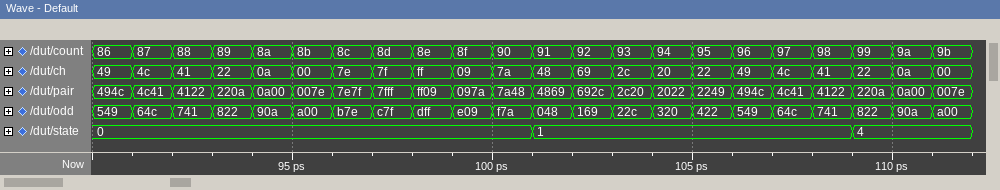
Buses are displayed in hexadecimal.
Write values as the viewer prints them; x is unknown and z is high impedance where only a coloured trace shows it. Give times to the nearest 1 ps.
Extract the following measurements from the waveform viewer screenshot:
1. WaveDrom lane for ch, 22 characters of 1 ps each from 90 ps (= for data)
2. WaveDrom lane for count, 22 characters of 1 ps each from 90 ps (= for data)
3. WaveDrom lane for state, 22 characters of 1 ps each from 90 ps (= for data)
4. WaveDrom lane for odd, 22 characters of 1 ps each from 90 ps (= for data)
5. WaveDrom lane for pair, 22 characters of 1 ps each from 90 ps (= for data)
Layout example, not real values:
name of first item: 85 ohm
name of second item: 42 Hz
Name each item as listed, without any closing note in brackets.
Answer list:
WaveDrom lane for ch, 22 characters of 1 ps each from 90 ps: {name: 'ch', wave: '======================', data: '49 4c 41 22 0a 00 7e 7f ff 09 7a 48 69 2c 20 22 49 4c 41 22 0a 00'}
WaveDrom lane for count, 22 characters of 1 ps each from 90 ps: {name: 'count', wave: '======================', data: '86 87 88 89 8a 8b 8c 8d 8e 8f 90 91 92 93 94 95 96 97 98 99 9a 9b'}
WaveDrom lane for state, 22 characters of 1 ps each from 90 ps: {name: 'state', wave: '=..........=.......=..', data: '0 1 4'}
WaveDrom lane for odd, 22 characters of 1 ps each from 90 ps: {name: 'odd', wave: '======================', data: '549 64c 741 822 90a a00 b7e c7f dff e09 f7a 048 169 22c 320 422 549 64c 741 822 90a a00'}
WaveDrom lane for pair, 22 characters of 1 ps each from 90 ps: {name: 'pair', wave: '======================', data: '494c 4c41 4122 220a 0a00 007e 7e7f 7fff ff09 097a 7a48 4869 692c 2c20 2022 2249 494c 4c41 4122 220a 0a00 007e'}
